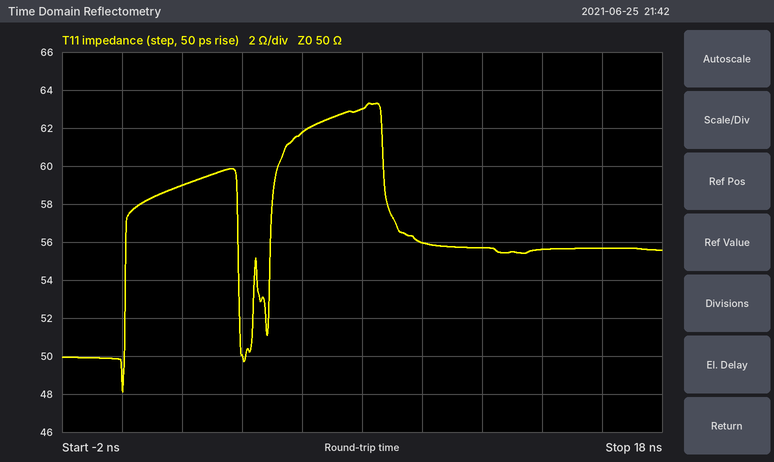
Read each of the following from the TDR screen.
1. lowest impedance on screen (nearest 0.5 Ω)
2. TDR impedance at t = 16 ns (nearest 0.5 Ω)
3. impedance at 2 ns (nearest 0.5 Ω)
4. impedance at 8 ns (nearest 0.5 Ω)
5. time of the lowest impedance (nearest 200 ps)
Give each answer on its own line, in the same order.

48.0 Ω
55.5 Ω
59.0 Ω
63.0 Ω
0.0 ns
